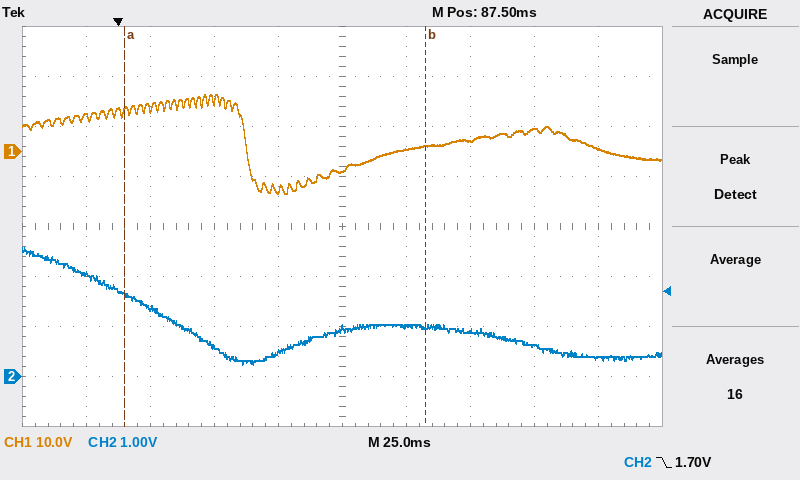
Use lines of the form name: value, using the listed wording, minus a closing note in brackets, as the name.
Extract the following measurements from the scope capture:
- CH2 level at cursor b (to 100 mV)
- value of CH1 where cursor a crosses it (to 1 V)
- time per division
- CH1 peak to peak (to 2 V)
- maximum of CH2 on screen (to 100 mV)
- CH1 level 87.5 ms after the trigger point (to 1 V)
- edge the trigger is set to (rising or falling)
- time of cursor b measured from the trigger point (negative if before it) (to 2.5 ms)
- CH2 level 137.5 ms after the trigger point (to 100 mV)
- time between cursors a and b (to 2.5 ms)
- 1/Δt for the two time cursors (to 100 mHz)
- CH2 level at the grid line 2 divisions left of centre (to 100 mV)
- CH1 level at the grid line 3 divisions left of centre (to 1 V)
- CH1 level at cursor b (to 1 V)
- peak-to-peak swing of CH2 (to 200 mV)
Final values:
CH2 level at cursor b: 1.0 V
value of CH1 where cursor a crosses it: 8 V
time per division: 25 ms
CH1 peak to peak: 20 V
maximum of CH2 on screen: 2.6 V
CH1 level 87.5 ms after the trigger point: -4 V
edge the trigger is set to: falling
time of cursor b measured from the trigger point (negative if before it): +120.0 ms
CH2 level 137.5 ms after the trigger point: 900 mV
time between cursors a and b: 117.5 ms
1/Δt for the two time cursors: 8.5 Hz
CH2 level at the grid line 2 divisions left of centre: 600 mV
CH1 level at the grid line 3 divisions left of centre: 9 V
CH1 level at cursor b: 1 V
peak-to-peak swing of CH2: 2.4 V
